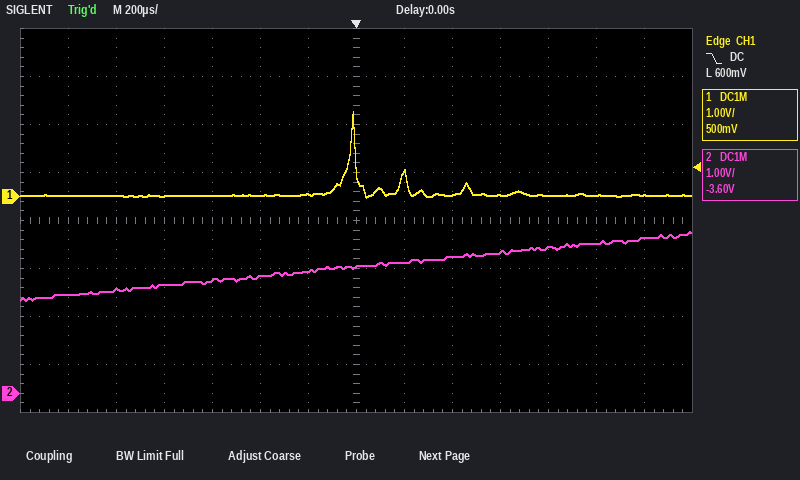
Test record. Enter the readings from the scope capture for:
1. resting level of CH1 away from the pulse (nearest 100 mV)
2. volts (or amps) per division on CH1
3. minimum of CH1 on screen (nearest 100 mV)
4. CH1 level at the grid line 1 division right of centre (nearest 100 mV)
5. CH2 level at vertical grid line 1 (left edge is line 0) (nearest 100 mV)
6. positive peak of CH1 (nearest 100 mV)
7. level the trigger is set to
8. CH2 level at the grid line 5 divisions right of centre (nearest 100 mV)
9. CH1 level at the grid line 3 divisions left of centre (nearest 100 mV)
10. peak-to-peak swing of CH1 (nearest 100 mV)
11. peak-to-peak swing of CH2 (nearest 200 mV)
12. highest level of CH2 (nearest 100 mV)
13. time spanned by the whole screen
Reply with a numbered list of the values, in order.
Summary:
1. 0.0 V
2. 1 V
3. 0.0 V
4. 500 mV
5. 2.1 V
6. 1.8 V
7. 600 mV
8. 3.1 V
9. 0.0 V
10. 1.8 V
11. 1.4 V
12. 3.4 V
13. 2.8 ms
